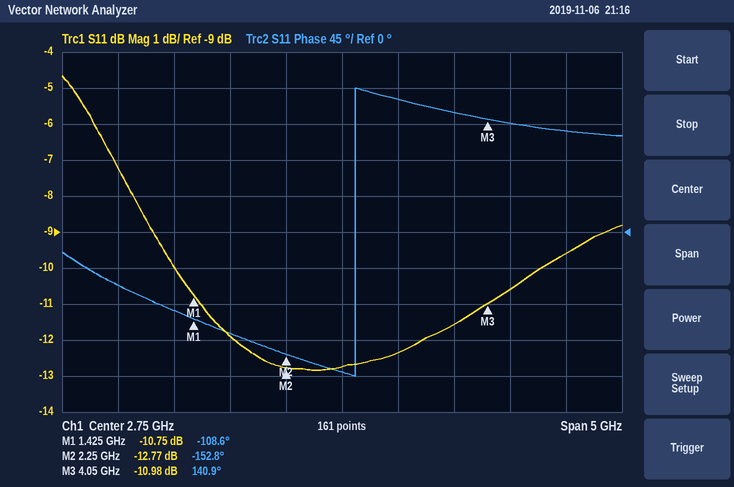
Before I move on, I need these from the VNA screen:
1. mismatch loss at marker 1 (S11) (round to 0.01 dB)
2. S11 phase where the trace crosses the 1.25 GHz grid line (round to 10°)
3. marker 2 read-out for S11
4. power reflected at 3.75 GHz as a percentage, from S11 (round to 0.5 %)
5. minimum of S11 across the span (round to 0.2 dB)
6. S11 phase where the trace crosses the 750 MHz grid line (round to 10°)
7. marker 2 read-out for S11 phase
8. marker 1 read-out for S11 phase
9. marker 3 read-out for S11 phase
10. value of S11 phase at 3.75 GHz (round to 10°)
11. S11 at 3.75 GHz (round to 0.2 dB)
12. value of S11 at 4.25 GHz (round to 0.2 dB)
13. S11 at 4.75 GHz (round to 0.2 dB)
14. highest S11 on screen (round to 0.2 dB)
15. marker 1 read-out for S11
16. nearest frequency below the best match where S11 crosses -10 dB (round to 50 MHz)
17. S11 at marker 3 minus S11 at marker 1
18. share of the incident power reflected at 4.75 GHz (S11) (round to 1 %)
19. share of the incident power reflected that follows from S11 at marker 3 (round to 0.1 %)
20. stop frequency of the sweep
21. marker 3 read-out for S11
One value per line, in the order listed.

0.38 dB
-100°
-12.77 dB
7.0 %
-12.8 dB
-70°
-152.8°
-108.6°
140.9°
150°
-11.6 dB
-10.6 dB
-9.6 dB
-4.6 dB
-10.75 dB
1.25 GHz
-0.23 dB
11 %
8.0 %
5.25 GHz
-10.98 dB
